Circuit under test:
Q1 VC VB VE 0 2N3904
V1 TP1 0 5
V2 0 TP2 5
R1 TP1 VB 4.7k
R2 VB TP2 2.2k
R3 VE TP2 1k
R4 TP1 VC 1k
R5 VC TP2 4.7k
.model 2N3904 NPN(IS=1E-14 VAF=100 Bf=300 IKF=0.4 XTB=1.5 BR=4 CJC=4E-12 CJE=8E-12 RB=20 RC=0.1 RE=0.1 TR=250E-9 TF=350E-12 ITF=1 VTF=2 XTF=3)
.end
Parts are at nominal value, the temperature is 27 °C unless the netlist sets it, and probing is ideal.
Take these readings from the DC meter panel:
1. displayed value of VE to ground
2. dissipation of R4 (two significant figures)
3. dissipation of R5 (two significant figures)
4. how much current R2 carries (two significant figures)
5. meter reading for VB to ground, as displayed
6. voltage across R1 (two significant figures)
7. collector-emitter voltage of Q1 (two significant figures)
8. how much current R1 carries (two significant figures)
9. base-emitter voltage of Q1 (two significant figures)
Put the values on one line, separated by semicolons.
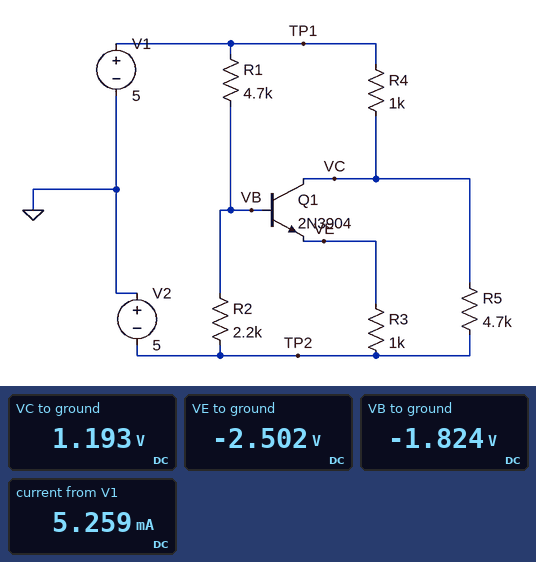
-2.502 V; 14 mW; 8.2 mW; 1.4 mA; -1.824 V; 6.8 V; 3.7 V; 1.5 mA; 680 mV
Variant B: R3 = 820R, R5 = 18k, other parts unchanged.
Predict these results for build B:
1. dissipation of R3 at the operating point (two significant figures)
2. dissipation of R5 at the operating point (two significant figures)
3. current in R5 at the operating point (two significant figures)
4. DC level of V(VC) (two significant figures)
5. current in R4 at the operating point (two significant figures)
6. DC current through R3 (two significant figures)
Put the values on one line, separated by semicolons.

7.6 mW; 2.4 mW; 370 µA; 1.6 V; 3.4 mA; 3.0 mA
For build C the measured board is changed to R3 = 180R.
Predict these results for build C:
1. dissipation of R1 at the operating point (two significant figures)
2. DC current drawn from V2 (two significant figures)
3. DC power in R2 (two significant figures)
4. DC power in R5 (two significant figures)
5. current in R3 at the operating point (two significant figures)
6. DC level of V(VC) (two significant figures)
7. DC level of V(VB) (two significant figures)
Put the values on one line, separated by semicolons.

13 mW; 10 mA; 2.4 mW; 550 µW; 8.7 mA; -3.4 V; -2.7 V
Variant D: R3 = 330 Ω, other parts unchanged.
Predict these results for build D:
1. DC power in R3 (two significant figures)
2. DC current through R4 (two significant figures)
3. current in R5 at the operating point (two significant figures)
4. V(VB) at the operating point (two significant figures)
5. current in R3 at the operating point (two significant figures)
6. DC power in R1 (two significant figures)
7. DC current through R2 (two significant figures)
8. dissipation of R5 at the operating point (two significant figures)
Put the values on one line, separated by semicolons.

17 mW; 7.6 mA; 520 µA; -1.9 V; 7.1 mA; 10 mW; 1.4 mA; 1.3 mW
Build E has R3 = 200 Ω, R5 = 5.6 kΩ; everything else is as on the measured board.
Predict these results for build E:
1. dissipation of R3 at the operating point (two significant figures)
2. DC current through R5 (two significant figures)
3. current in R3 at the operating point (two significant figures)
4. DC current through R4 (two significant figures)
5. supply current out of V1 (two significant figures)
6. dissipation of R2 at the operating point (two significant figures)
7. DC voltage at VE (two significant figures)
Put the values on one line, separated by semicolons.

14 mW; 310 µA; 8.5 mA; 8.3 mA; 9.9 mA; 2.7 mW; -3.3 V
